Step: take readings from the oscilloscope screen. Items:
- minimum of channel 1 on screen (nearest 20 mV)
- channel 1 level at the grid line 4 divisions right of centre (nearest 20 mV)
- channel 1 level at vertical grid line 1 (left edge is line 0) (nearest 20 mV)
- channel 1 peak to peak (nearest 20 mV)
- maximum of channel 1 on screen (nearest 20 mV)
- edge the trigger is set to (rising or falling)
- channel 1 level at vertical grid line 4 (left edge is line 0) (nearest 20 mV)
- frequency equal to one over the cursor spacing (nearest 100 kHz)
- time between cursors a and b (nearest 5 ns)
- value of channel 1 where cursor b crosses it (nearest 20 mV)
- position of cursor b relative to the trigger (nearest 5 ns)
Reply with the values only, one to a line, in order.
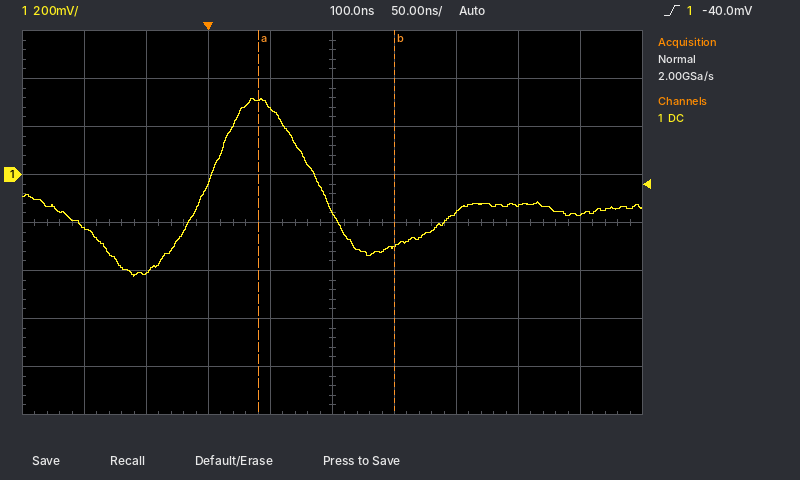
-420 mV
-160 mV
-220 mV
740 mV
320 mV
rising
280 mV
9.1 MHz
110 ns
-300 mV
+150 ns
